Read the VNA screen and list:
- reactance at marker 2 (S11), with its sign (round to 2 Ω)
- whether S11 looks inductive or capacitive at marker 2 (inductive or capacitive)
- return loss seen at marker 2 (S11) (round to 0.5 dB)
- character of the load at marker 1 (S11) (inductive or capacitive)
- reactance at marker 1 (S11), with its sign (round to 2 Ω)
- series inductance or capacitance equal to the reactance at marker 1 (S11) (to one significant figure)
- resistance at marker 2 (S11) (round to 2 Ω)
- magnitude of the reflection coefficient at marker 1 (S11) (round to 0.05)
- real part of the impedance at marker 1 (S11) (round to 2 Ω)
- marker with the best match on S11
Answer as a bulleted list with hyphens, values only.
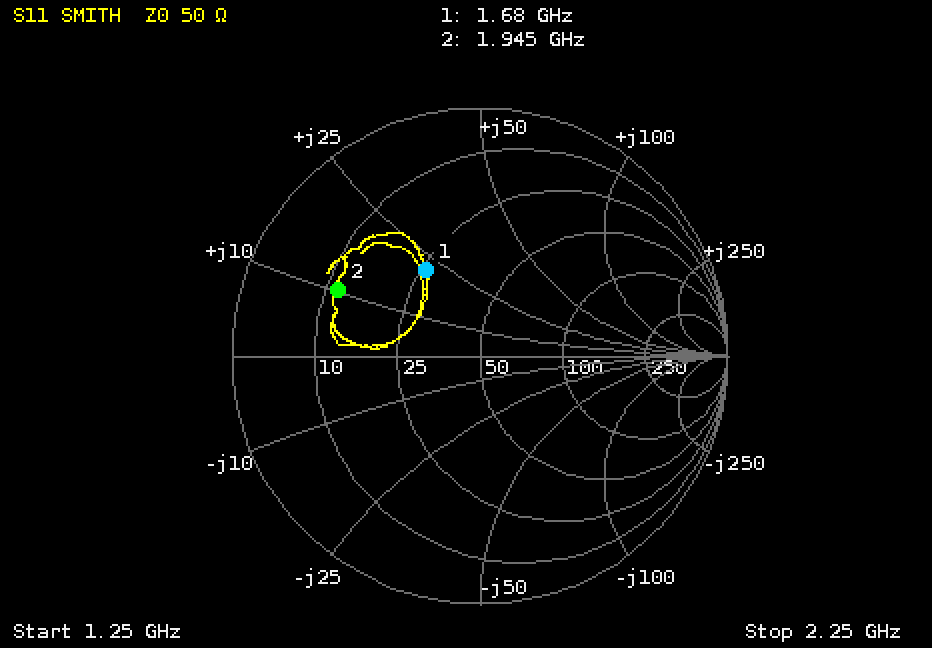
- +10 Ω
- inductive
- 4.0 dB
- inductive
- +22 Ω
- 2 nH
- 12 Ω
- 0.40
- 26 Ω
- marker 1
